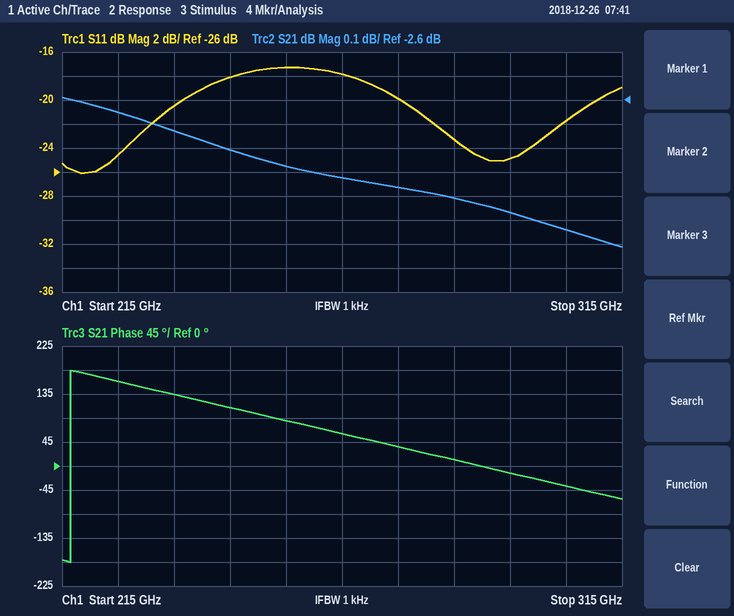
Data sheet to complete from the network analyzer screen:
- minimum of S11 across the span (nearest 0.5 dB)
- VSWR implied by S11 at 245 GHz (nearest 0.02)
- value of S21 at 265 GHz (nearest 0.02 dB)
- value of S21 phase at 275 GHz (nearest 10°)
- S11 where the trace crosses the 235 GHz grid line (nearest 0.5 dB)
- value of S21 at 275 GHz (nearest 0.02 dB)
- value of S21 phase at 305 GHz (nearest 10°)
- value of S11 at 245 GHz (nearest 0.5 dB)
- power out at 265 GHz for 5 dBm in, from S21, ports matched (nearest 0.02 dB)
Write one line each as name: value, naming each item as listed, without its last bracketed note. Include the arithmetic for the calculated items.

minimum of S11 across the span: -26.0 dB
VSWR implied by S11 at 245 GHz: |Γ| = 10^(-18/20) = 0.1259; VSWR = (1 + 0.1259)/(1 − 0.1259) ≈ 1.29, so 1.28 to the nearest 0.02
value of S21 at 265 GHz: -2.92 dB
value of S21 phase at 275 GHz: 40°
S11 where the trace crosses the 235 GHz grid line: -20.5 dB
value of S21 at 275 GHz: -2.96 dB
value of S21 phase at 305 GHz: -40°
value of S11 at 245 GHz: -18.0 dB
power out at 265 GHz for 5 dBm in, from S21, ports matched: 5 dBm + (-2.92 dB) = 2.08 dBm
